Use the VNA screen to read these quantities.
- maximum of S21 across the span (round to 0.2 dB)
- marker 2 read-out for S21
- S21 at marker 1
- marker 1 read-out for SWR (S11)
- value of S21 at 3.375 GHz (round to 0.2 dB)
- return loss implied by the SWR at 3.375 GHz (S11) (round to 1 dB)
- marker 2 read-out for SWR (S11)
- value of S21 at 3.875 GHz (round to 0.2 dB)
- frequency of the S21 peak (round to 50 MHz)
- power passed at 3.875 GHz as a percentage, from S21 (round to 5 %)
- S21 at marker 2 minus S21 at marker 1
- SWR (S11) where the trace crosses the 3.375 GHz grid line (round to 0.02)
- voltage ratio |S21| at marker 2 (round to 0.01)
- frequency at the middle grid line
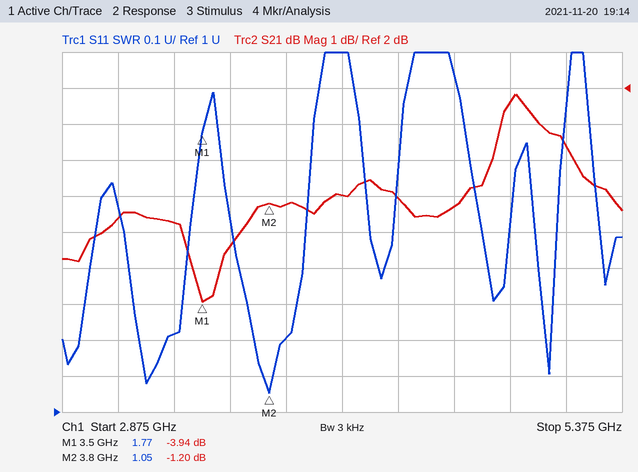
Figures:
1.8 dB
-1.20 dB
-3.94 dB
1.77
-1.8 dB
20 dB
1.05
-1.2 dB
4.90 GHz
75 %
2.74 dB
1.22
0.87
4.125 GHz
